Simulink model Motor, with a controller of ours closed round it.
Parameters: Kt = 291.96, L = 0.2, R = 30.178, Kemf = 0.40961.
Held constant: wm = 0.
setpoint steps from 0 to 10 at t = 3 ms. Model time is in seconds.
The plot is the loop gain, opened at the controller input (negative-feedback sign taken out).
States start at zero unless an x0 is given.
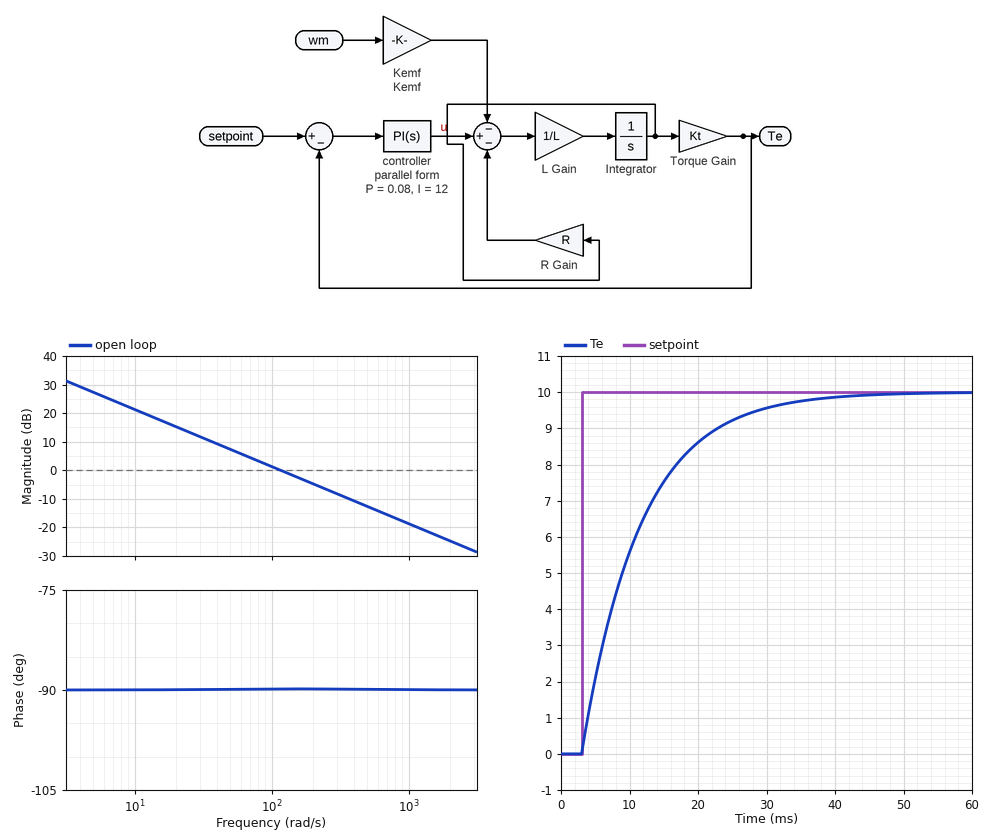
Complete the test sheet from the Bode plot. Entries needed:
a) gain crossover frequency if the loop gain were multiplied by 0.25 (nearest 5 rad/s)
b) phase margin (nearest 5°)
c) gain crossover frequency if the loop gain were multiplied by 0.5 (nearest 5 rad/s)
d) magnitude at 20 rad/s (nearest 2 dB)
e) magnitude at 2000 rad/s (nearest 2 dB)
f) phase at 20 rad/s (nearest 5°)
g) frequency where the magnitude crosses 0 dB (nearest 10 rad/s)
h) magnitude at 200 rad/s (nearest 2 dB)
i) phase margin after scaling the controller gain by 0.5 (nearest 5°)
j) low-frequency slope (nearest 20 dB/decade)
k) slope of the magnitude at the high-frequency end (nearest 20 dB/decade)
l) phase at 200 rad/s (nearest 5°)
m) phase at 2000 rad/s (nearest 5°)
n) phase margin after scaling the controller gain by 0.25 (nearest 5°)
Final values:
30 rad/s
90°
60 rad/s
16 dB
-24 dB
-90°
120 rad/s
-4 dB
90°
-20 dB/decade
-20 dB/decade
-90°
-90°
90°
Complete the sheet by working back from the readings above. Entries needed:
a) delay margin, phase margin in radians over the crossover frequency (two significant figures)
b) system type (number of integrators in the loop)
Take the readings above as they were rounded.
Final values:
0.013 s
1
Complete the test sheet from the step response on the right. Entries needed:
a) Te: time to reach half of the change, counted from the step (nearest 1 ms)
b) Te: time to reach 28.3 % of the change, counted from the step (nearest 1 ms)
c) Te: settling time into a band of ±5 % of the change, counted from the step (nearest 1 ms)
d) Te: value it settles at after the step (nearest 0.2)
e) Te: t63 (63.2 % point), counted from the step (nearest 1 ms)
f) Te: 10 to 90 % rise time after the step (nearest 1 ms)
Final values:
6 ms
3 ms
26 ms
10.0
9 ms
19 ms
